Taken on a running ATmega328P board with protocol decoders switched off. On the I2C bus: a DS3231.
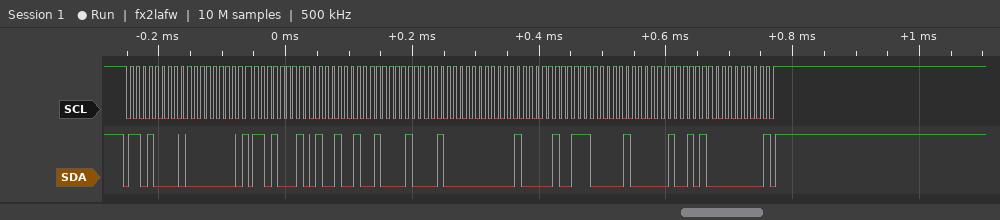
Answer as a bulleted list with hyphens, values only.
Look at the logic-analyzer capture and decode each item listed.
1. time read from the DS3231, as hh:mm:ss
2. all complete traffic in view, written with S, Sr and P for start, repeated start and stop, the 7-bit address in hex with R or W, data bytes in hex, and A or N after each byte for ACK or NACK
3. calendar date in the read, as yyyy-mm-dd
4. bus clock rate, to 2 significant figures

- 20:42:49
- S 68W A 00 A Sr 68R A 49 A 42 A 20 A 04 A 27 A 08 A 25 A 00 N P
- 2025-08-27
- 100 kHz
